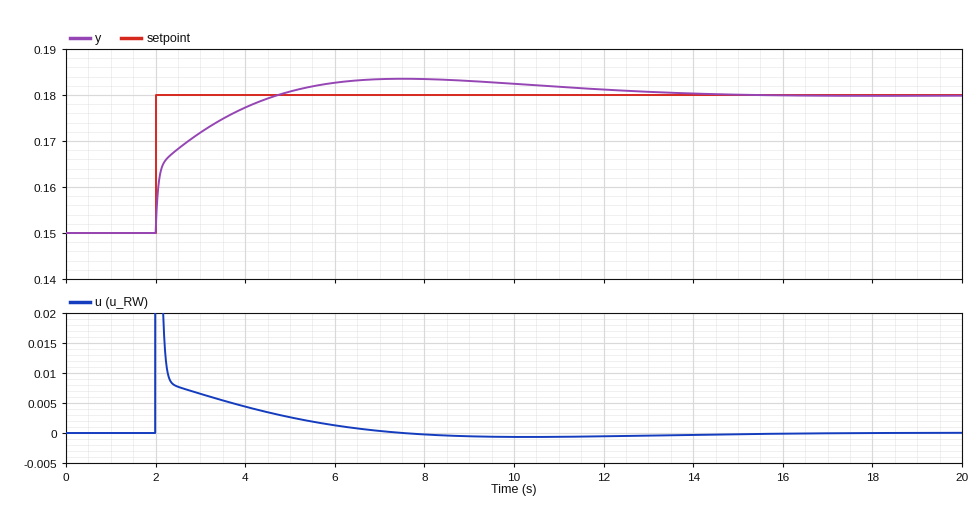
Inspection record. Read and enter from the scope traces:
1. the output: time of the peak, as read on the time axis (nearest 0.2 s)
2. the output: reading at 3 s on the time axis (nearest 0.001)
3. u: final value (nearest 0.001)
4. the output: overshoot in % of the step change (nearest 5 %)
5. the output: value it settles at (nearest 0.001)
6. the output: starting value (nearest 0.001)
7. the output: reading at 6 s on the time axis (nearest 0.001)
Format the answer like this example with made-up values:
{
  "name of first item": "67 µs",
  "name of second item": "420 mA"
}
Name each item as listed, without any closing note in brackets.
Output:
{
  "the output: time of the peak, as read on the time axis": "7.6 s",
  "the output: reading at 3 s on the time axis": "0.172",
  "u: final value": "0.000",
  "the output: overshoot in % of the step change": "10 %",
  "the output: value it settles at": "0.180",
  "the output: starting value": "0.150",
  "the output: reading at 6 s on the time axis": "0.183"
}
